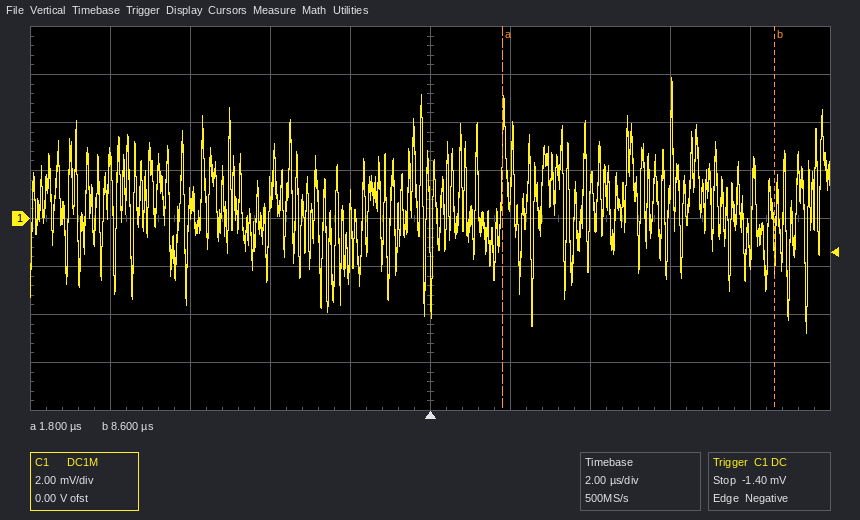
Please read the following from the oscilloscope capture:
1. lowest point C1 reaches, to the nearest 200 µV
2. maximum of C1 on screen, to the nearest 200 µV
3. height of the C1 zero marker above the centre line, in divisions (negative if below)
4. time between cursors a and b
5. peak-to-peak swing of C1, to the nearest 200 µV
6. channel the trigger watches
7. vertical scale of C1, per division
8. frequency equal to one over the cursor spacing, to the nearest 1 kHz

-4.8 mV
5.8 mV
0.0 div
6.8 µs
10.6 mV
C1
2 mV
147 kHz
